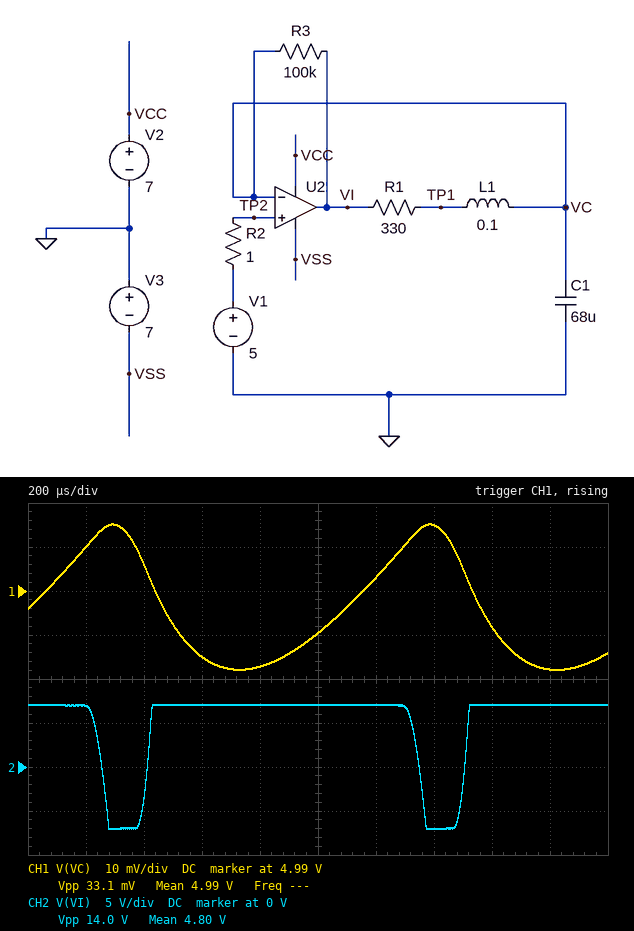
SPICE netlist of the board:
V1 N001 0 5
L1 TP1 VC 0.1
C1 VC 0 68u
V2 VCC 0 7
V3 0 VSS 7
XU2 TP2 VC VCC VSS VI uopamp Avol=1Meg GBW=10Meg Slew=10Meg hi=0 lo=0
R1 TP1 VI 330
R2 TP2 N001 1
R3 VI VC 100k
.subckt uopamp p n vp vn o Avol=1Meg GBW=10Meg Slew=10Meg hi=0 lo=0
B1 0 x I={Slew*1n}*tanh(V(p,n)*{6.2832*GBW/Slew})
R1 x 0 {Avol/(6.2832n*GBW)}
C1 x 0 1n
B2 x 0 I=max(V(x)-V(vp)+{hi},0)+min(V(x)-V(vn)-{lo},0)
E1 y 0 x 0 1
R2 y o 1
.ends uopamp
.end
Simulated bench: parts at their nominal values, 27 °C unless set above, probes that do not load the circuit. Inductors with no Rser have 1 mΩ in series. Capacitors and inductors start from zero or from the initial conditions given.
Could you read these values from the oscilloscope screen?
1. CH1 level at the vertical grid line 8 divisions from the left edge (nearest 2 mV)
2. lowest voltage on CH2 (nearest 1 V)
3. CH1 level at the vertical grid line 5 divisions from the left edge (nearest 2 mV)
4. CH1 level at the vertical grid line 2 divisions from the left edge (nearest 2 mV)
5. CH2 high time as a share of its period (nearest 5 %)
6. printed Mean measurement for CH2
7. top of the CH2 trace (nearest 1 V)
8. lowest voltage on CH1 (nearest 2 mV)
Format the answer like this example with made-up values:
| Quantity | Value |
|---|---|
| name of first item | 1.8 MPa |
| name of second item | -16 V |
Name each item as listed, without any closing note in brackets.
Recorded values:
| Quantity | Value |
|---|---|
| CH1 level at the vertical grid line 8 divisions from the left edge | 4.982 V |
| lowest voltage on CH2 | -7 V |
| CH1 level at the vertical grid line 5 divisions from the left edge | 4.980 V |
| CH1 level at the vertical grid line 2 divisions from the left edge | 4.996 V |
| CH2 high time as a share of its period | 85 % |
| printed Mean measurement for CH2 | 4.80 V |
| top of the CH2 trace | 7 V |
| lowest voltage on CH1 | 4.972 V |
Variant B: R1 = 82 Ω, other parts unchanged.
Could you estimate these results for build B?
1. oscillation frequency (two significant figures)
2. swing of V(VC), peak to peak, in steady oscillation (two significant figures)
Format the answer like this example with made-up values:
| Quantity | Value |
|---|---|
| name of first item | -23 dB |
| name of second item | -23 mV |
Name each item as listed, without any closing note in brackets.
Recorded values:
| Quantity | Value |
|---|---|
| oscillation frequency | 560 Hz |
| swing of V(VC), peak to peak, in steady oscillation | 100 mV |
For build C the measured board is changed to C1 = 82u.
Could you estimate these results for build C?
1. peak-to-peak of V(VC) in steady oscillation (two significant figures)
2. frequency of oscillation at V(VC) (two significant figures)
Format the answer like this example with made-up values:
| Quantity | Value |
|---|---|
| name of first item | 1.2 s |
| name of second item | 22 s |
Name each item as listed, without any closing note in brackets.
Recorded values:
| Quantity | Value |
|---|---|
| peak-to-peak of V(VC) in steady oscillation | 30 mV |
| frequency of oscillation at V(VC) | 870 Hz |
